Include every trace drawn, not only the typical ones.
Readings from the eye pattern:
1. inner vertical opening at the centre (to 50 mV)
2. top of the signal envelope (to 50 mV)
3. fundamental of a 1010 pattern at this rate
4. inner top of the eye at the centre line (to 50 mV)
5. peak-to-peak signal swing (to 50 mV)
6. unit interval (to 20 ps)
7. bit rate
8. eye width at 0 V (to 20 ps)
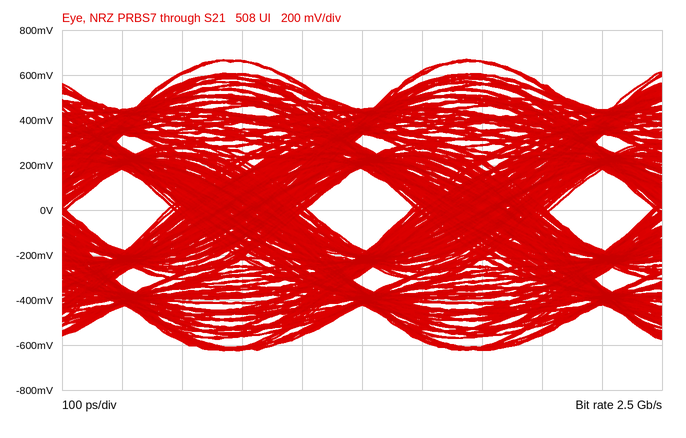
350 mV
650 mV
1.25 GHz
200 mV
1.30 V
400 ps
2.5 Gb/s
180 ps
